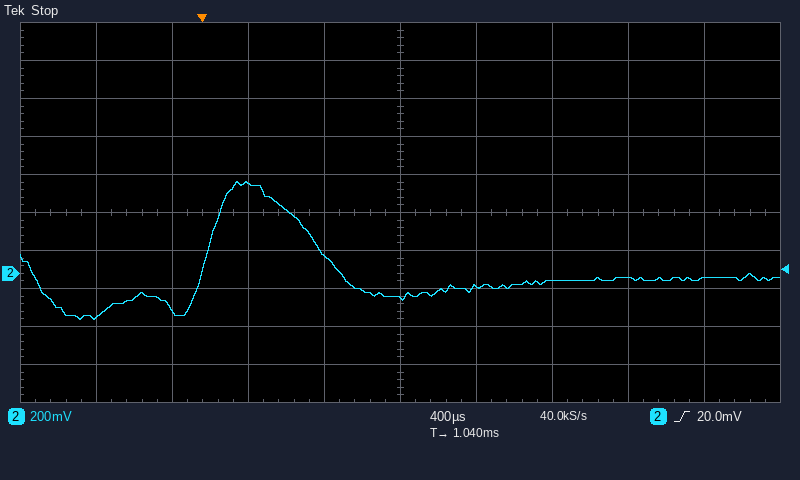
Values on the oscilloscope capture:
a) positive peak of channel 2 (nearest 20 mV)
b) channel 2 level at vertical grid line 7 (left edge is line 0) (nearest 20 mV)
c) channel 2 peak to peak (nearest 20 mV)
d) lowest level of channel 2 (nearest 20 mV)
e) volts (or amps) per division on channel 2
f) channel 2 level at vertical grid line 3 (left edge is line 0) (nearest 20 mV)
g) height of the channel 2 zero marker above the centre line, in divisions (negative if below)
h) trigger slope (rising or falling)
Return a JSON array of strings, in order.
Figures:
["480 mV", "-40 mV", "720 mV", "-240 mV", "200 mV", "480 mV", "-1.6 div", "rising"]
